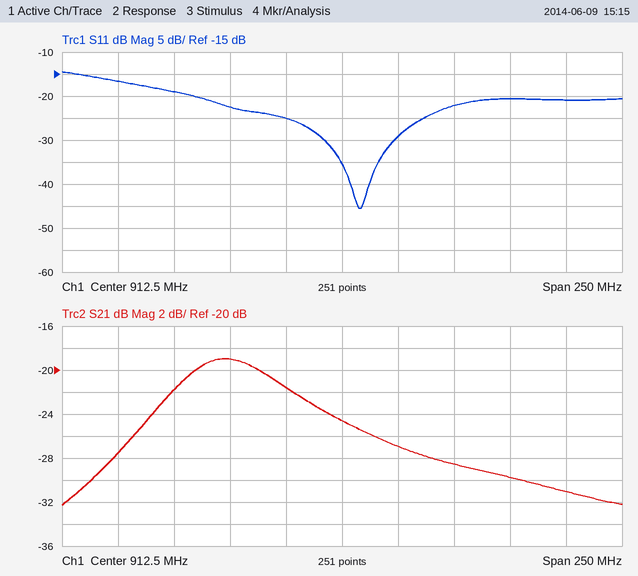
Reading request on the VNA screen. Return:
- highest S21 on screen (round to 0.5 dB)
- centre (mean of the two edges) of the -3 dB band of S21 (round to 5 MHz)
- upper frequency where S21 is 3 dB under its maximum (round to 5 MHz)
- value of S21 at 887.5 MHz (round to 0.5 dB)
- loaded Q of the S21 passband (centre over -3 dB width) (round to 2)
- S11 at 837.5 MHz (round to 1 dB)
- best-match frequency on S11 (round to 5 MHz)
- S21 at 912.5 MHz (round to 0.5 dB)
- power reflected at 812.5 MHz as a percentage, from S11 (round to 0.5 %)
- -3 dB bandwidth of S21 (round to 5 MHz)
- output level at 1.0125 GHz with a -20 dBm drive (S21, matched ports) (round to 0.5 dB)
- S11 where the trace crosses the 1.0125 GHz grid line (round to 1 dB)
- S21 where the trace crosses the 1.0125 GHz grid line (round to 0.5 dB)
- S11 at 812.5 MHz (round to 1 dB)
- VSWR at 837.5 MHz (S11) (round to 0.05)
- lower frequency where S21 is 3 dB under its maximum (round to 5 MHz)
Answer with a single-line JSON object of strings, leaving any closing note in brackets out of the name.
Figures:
{"highest S21 on screen": "-19.0 dB", "centre (mean of the two edges) of the -3 dB band of S21": "865 MHz", "upper frequency where S21 is 3 dB under its maximum": "890 MHz", "value of S21 at 887.5 MHz": "-21.5 dB", "loaded Q of the S21 passband (centre over -3 dB width)": "16", "S11 at 837.5 MHz": "-19 dB", "best-match frequency on S11": "920 MHz", "S21 at 912.5 MHz": "-24.5 dB", "power reflected at 812.5 MHz as a percentage, from S11": "2.0 %", "-3 dB bandwidth of S21": "55 MHz", "output level at 1.0125 GHz with a -20 dBm drive (S21, matched ports)": "-51.0 dBm", "S11 where the trace crosses the 1.0125 GHz grid line": "-21 dB", "S21 where the trace crosses the 1.0125 GHz grid line": "-31.0 dB", "S11 at 812.5 MHz": "-17 dB", "VSWR at 837.5 MHz (S11)": "1.25", "lower frequency where S21 is 3 dB under its maximum": "835 MHz"}
